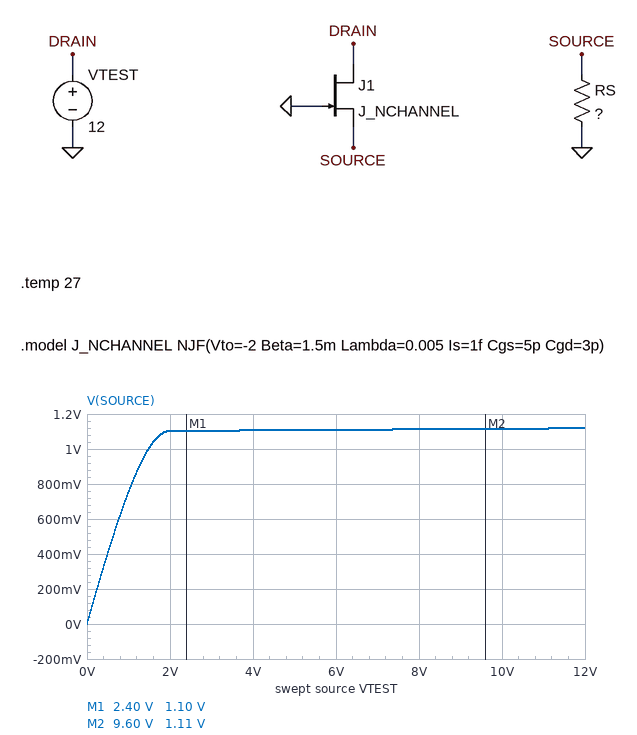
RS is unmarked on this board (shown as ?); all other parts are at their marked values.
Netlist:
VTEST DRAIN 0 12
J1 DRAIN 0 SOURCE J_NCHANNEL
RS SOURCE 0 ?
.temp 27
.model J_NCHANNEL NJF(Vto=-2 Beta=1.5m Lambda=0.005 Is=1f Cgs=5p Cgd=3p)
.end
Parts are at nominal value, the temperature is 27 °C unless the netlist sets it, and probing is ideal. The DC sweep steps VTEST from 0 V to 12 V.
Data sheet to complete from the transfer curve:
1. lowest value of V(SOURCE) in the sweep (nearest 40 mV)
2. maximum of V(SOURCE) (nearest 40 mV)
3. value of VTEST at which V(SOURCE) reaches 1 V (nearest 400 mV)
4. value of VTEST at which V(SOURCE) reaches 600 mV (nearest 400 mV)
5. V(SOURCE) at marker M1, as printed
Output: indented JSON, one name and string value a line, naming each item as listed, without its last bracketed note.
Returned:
{
  "lowest value of V(SOURCE) in the sweep": "0 V",
  "maximum of V(SOURCE)": "1.12 V",
  "value of VTEST at which V(SOURCE) reaches 1 V": "1.6 V",
  "value of VTEST at which V(SOURCE) reaches 600 mV": "800 mV",
  "V(SOURCE) at marker M1, as printed": "1.10 V"
}
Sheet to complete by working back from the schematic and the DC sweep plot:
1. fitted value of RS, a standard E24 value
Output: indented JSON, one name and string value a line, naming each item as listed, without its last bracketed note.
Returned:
{
  "fitted value of RS, a standard E24 value": "910 Ω"
}
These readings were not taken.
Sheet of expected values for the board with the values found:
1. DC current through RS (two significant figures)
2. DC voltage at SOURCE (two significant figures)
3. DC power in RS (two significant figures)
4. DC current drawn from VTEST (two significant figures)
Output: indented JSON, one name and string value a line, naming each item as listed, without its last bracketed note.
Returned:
{
  "DC current through RS": "1.2 mA",
  "DC voltage at SOURCE": "1.1 V",
  "DC power in RS": "1.4 mW",
  "DC current drawn from VTEST": "1.2 mA"
}
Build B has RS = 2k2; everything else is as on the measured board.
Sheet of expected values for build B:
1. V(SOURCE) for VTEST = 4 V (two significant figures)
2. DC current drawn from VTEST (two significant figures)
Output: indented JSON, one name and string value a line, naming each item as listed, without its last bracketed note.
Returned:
{
  "V(SOURCE) for VTEST = 4 V": "1.4 V",
  "DC current drawn from VTEST": "620 µA"
}
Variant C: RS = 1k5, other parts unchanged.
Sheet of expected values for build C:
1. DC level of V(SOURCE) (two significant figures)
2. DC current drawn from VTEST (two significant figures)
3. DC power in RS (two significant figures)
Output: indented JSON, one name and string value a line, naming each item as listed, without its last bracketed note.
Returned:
{
  "DC level of V(SOURCE)": "1.3 V",
  "DC current drawn from VTEST": "850 µA",
  "DC power in RS": "1.1 mW"
}
